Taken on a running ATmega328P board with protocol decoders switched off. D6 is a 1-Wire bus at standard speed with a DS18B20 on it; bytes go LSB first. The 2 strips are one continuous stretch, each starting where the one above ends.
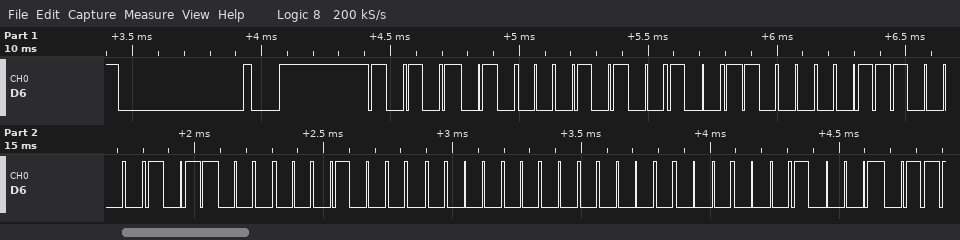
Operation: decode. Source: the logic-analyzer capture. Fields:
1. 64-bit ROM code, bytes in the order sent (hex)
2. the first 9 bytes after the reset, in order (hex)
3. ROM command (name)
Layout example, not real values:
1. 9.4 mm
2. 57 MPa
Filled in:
1. 28 19 1C 1A 08 00 00 88
2. 55 28 19 1C 1A 08 00 00 88
3. Match ROM
